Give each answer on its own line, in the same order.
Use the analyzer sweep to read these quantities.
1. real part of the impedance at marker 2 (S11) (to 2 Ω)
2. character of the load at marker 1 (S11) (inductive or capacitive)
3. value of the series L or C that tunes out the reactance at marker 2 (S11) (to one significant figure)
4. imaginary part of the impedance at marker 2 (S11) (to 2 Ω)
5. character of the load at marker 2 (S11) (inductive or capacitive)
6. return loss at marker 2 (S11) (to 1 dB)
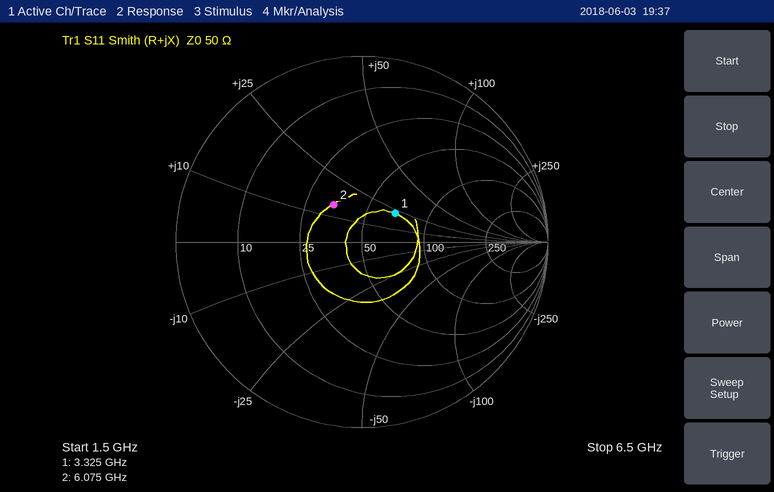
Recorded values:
34 Ω
inductive
2 pF
+14 Ω
inductive
12 dB
